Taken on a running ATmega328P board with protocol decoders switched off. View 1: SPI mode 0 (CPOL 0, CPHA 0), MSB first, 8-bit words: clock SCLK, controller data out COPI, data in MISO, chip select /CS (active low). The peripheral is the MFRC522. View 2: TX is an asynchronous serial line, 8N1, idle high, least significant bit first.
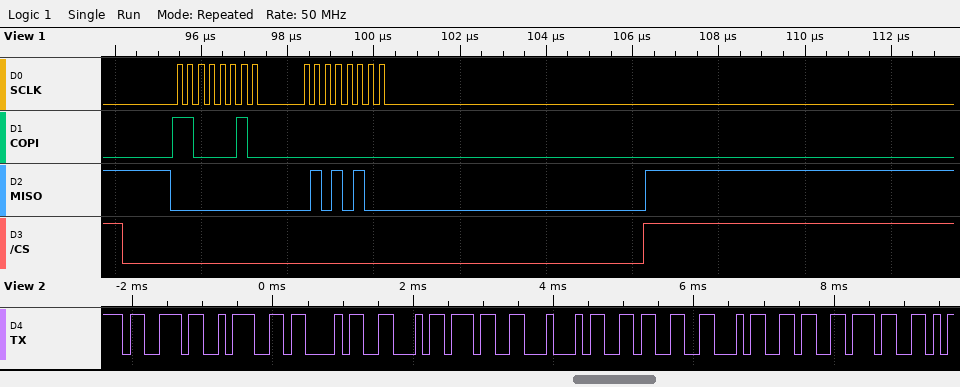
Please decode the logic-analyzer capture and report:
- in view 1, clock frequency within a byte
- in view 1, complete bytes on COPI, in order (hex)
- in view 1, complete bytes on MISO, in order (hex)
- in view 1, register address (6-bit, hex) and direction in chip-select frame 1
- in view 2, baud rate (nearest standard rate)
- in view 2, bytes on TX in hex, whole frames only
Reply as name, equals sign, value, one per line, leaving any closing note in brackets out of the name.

in view 1, clock frequency within a byte = 4 MHz
in view 1, complete bytes on COPI, in order = C2 00
in view 1, complete bytes on MISO, in order = 00 54
in view 1, register address (6-bit, hex) and direction in chip-select frame 1 = 0x21 read
in view 2, baud rate = 9600 baud
in view 2, bytes on TX in hex, whole frames only = 0x73 0x3A 0x43 0x46 0x37 0x44 0x36 0x46 0x36 0x37
